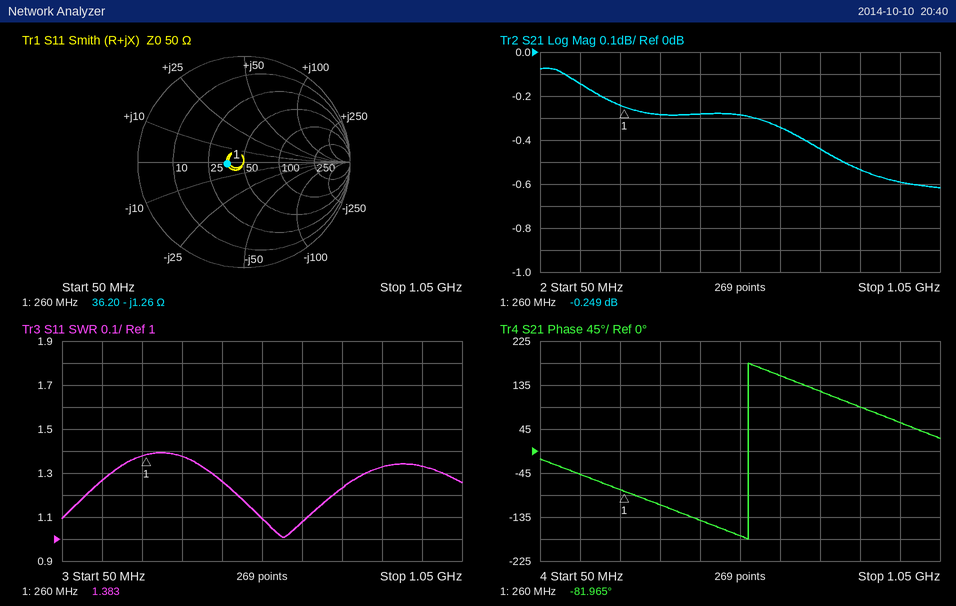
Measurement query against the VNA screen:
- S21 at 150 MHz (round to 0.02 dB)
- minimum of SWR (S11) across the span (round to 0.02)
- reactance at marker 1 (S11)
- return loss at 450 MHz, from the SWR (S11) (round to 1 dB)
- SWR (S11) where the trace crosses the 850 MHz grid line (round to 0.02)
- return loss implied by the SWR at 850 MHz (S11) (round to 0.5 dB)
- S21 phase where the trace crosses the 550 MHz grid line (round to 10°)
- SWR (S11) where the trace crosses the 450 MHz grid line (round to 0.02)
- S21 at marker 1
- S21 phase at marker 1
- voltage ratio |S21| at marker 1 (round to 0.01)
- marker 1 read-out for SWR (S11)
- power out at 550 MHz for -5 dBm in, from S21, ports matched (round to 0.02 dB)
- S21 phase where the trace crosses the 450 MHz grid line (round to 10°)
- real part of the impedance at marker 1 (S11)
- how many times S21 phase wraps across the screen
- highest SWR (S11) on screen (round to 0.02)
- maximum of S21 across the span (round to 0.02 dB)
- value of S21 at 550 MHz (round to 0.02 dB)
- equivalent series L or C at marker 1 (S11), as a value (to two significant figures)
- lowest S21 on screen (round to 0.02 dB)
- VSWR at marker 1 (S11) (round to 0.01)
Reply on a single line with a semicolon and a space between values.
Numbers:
-0.14 dB; 1.00; -1.26 Ω; 19 dB; 1.32; 17.0 dB; -170°; 1.26; -0.249 dB; -81.965°; 0.97; 1.383; -5.28 dBm; -140°; 36.20 Ω; 1; 1.40; -0.08 dB; -0.28 dB; 490 pF; -0.62 dB; 1.38
